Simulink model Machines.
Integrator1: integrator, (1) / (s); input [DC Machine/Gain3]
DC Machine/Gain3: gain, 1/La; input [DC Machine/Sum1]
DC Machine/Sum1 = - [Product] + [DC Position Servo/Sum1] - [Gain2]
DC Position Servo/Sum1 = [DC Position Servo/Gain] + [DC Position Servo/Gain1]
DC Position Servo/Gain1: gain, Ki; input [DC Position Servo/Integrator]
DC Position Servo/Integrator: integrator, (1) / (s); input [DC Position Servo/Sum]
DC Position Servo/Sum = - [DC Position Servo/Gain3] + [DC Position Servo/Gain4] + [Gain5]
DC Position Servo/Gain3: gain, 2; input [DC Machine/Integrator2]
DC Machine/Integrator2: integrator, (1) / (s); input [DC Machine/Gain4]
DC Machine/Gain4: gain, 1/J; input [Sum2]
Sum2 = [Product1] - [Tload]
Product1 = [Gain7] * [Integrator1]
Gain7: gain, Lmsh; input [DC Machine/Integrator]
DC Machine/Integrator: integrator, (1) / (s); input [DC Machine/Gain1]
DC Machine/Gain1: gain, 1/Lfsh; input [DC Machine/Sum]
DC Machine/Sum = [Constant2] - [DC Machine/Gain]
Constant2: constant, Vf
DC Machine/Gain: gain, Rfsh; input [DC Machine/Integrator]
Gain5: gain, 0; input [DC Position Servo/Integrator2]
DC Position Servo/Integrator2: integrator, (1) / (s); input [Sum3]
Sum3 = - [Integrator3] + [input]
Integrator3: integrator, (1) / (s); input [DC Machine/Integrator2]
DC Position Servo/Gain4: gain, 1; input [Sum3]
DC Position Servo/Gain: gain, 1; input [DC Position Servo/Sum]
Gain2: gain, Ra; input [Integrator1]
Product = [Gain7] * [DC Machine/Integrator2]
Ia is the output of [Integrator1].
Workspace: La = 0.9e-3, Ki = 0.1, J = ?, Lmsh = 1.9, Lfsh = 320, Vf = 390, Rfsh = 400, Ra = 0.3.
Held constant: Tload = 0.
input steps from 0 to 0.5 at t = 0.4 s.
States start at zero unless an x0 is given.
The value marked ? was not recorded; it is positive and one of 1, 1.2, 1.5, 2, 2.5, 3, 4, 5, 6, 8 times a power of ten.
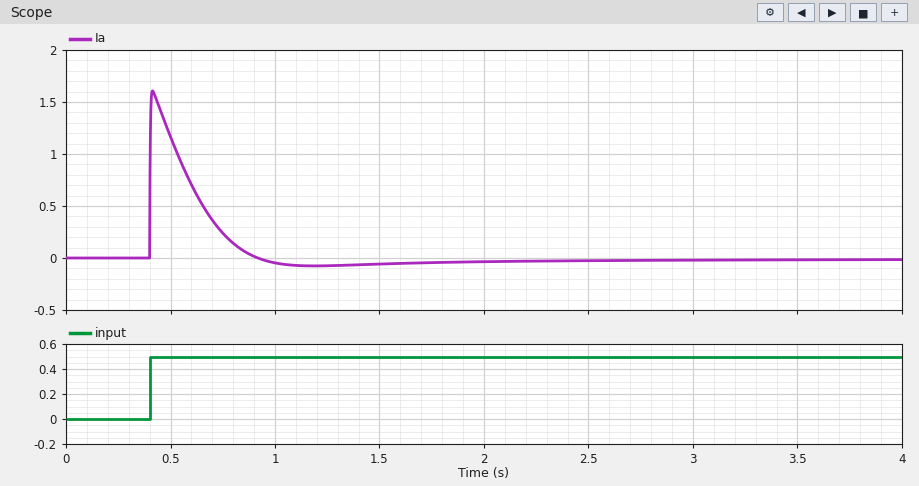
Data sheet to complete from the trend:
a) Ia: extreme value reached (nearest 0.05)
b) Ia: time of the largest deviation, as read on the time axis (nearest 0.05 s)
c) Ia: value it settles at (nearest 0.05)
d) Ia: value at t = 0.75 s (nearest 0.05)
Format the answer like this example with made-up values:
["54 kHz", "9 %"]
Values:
["1.60", "0.40 s", "0.00", "0.25"]
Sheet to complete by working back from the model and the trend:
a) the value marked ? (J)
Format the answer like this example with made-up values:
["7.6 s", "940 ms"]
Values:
["2"]
